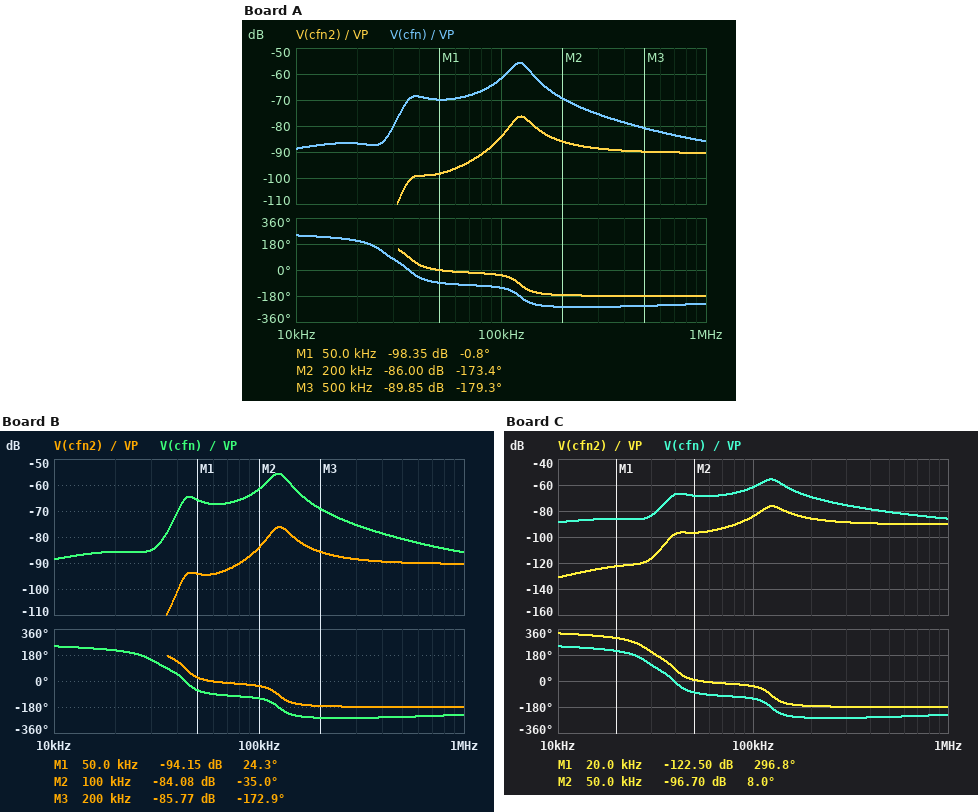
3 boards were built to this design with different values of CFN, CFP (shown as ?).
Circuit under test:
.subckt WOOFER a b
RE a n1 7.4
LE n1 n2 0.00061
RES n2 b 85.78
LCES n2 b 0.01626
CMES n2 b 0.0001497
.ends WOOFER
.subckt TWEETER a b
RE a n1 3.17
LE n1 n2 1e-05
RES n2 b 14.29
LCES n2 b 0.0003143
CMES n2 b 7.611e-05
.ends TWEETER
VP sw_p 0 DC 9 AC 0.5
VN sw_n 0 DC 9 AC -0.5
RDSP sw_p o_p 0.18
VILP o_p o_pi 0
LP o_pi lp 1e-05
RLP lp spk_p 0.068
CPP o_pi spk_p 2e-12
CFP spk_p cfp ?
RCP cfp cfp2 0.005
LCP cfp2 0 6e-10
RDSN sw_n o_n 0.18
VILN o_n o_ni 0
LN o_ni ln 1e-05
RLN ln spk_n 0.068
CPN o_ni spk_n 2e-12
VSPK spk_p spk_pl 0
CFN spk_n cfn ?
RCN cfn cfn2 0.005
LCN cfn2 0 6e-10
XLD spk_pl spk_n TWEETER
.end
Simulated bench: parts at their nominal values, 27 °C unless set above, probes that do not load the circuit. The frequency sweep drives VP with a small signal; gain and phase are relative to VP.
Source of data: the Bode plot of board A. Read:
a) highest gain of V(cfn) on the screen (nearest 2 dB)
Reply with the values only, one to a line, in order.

-56 dB
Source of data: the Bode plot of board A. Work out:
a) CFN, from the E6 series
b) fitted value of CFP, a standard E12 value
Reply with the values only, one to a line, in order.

330 nF
2.7 µF
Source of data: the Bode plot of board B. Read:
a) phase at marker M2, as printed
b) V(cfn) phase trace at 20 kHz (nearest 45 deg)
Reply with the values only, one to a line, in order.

-35.0 deg
225 deg
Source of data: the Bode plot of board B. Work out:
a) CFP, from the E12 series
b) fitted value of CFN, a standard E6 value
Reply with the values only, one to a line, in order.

1.8 µF
330 nF
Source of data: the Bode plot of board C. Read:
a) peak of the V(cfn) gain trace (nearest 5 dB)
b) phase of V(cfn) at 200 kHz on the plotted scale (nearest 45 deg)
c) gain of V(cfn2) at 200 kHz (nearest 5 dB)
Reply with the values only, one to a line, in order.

-55 dB
-270 deg
-85 dB
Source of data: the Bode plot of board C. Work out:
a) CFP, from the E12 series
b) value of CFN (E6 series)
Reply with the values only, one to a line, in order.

2.2 µF
330 nF
